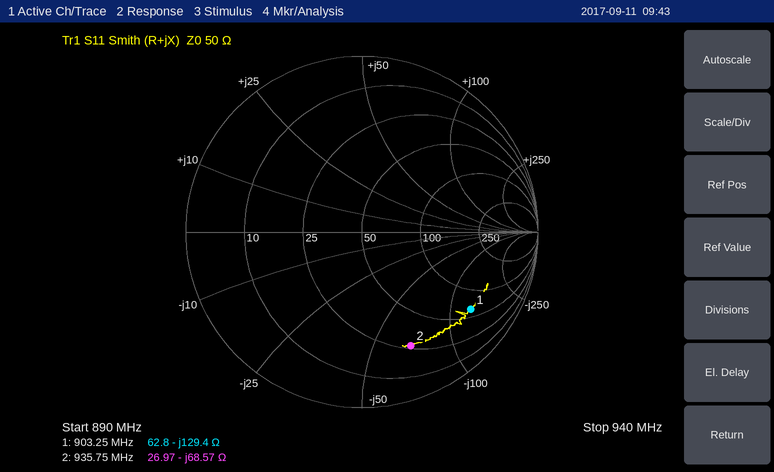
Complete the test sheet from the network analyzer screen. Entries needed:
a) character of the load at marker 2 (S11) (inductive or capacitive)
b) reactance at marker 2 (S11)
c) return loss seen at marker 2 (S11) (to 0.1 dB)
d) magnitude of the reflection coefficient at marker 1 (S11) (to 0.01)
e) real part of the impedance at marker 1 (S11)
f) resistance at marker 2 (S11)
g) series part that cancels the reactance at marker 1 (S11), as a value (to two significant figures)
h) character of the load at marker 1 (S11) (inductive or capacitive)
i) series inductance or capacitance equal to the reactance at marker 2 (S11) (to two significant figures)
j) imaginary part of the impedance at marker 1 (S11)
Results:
capacitive
-68.57 Ω
3.1 dB
0.76
62.8 Ω
26.97 Ω
23 nH
capacitive
2.5 pF
-129.4 Ω
